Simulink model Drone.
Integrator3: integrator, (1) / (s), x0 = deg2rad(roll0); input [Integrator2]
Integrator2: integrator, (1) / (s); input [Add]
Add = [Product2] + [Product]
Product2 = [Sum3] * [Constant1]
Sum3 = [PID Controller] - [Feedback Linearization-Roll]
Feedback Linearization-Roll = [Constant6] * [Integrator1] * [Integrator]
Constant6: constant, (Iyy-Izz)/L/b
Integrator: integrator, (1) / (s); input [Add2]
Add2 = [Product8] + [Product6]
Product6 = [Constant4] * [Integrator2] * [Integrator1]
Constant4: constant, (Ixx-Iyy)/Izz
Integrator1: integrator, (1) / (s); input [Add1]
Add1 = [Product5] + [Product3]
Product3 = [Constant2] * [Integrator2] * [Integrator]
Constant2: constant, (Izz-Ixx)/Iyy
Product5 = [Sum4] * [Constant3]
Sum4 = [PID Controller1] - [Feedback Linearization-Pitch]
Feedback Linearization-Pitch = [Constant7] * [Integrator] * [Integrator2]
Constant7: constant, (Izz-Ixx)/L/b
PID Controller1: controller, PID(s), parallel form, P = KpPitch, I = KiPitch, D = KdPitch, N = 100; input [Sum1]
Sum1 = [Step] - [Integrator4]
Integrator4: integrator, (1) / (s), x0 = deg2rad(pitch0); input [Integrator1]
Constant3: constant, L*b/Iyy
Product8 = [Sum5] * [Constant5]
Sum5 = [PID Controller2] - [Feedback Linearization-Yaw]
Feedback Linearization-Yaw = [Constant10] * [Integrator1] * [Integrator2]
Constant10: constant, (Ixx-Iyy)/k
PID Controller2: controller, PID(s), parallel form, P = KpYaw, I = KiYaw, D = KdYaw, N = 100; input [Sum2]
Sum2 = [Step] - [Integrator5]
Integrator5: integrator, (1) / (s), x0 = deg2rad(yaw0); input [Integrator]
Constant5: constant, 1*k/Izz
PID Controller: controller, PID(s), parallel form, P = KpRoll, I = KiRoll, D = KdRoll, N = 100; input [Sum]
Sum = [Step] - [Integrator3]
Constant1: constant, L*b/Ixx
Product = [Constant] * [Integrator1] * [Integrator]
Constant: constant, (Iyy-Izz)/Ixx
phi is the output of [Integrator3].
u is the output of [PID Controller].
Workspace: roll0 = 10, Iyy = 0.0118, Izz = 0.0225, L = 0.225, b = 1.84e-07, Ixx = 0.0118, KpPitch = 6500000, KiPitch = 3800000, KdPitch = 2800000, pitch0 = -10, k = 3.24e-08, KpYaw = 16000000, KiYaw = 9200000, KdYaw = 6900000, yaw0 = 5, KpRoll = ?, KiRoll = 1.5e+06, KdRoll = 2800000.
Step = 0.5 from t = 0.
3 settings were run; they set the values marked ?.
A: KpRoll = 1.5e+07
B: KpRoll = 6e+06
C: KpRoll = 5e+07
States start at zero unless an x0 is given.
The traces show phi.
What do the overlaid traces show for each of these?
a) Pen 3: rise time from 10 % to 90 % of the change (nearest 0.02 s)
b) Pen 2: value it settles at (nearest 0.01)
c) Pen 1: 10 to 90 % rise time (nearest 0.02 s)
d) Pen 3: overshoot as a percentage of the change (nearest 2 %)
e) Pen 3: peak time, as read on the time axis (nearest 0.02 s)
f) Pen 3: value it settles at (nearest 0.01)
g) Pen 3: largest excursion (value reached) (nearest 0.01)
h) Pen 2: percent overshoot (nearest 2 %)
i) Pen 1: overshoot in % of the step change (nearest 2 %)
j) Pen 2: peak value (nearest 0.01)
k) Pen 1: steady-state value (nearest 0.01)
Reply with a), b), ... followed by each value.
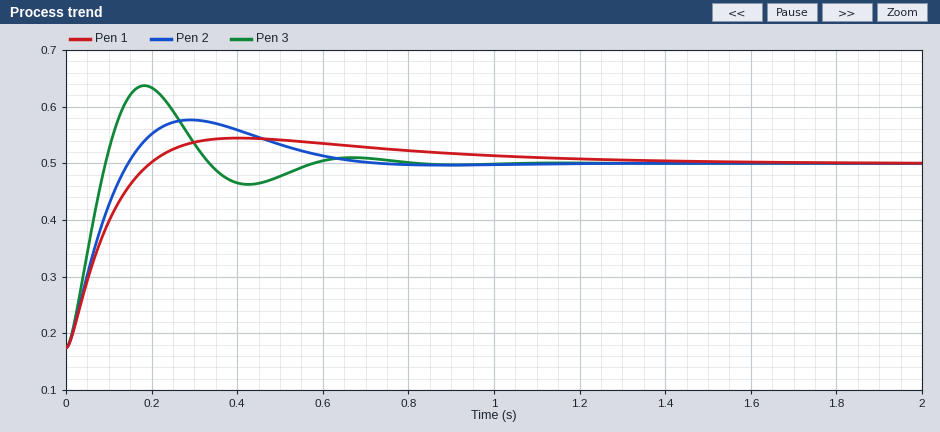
a) 0.06 s
b) 0.50
c) 0.14 s
d) 42 %
e) 0.18 s
f) 0.50
g) 0.64
h) 24 %
i) 14 %
j) 0.58
k) 0.50
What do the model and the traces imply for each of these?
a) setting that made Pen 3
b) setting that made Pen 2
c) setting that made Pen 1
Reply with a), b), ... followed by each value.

a) C
b) A
c) B
